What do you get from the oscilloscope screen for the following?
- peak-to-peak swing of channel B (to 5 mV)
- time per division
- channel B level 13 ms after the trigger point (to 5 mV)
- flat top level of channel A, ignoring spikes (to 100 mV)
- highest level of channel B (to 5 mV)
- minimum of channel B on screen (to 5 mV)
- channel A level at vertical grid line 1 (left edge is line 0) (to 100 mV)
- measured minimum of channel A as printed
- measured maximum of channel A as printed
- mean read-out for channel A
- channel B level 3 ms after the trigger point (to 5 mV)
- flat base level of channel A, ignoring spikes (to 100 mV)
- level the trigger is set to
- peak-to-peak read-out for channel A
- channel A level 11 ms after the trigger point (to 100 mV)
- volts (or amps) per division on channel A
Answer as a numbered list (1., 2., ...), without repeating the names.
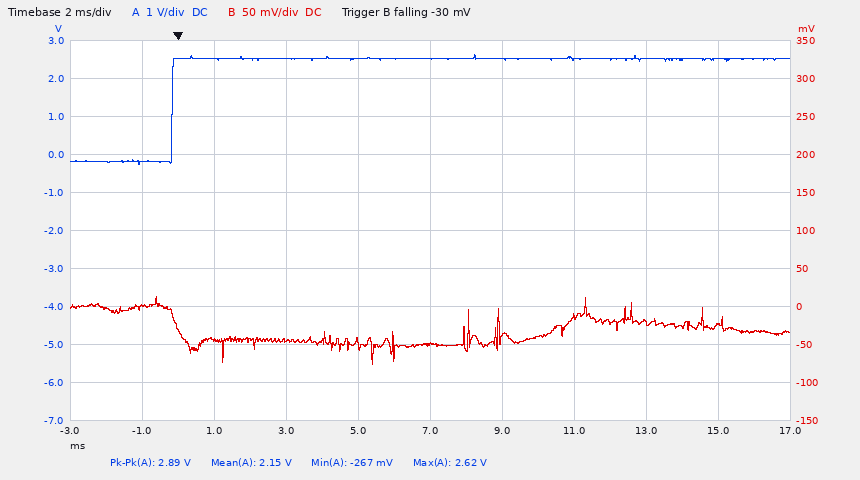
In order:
1. 90 mV
2. 2 ms
3. -20 mV
4. 2.5 V
5. 15 mV
6. -75 mV
7. -200 mV
8. -267 mV
9. 2.62 V
10. 2.15 V
11. -45 mV
12. -200 mV
13. -30 mV
14. 2.89 V
15. 2.5 V
16. 1 V
